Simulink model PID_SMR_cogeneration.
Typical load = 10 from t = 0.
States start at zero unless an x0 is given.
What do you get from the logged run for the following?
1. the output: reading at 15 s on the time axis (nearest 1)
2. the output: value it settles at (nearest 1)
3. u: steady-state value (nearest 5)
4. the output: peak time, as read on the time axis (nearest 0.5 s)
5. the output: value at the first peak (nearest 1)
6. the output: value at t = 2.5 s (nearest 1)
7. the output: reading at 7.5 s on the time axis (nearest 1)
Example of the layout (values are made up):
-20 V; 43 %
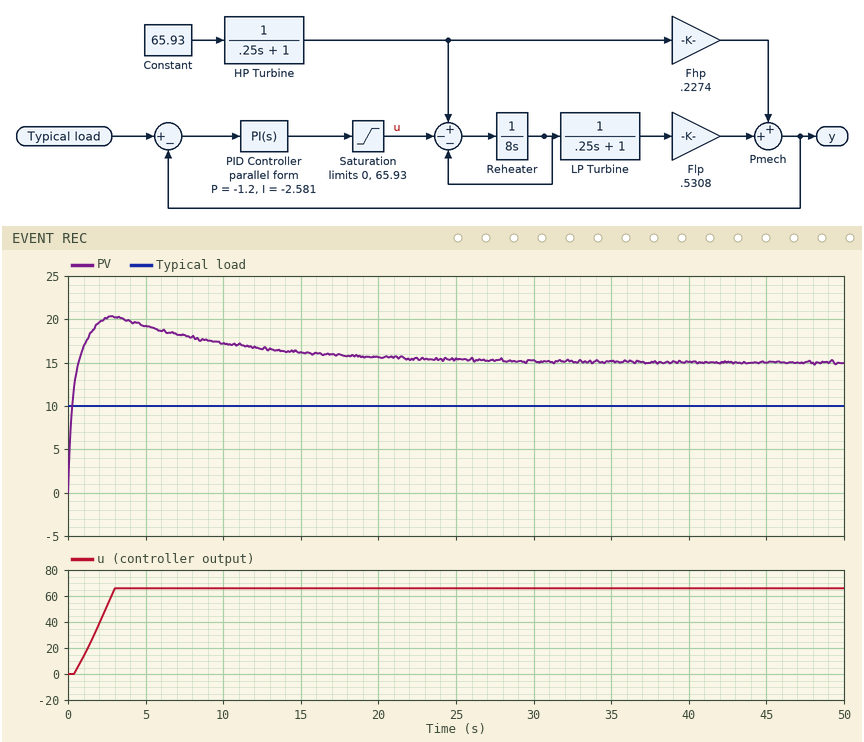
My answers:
16; 15; 65; 3.0 s; 20; 20; 18
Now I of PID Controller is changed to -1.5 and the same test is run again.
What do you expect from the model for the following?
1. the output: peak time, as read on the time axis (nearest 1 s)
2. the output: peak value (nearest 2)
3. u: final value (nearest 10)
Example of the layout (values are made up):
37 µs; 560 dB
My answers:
4 s; 22; 70
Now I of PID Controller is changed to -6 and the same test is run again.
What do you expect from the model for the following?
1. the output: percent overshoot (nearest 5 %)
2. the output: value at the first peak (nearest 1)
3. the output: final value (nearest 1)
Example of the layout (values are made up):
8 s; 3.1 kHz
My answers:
25 %; 19; 15
